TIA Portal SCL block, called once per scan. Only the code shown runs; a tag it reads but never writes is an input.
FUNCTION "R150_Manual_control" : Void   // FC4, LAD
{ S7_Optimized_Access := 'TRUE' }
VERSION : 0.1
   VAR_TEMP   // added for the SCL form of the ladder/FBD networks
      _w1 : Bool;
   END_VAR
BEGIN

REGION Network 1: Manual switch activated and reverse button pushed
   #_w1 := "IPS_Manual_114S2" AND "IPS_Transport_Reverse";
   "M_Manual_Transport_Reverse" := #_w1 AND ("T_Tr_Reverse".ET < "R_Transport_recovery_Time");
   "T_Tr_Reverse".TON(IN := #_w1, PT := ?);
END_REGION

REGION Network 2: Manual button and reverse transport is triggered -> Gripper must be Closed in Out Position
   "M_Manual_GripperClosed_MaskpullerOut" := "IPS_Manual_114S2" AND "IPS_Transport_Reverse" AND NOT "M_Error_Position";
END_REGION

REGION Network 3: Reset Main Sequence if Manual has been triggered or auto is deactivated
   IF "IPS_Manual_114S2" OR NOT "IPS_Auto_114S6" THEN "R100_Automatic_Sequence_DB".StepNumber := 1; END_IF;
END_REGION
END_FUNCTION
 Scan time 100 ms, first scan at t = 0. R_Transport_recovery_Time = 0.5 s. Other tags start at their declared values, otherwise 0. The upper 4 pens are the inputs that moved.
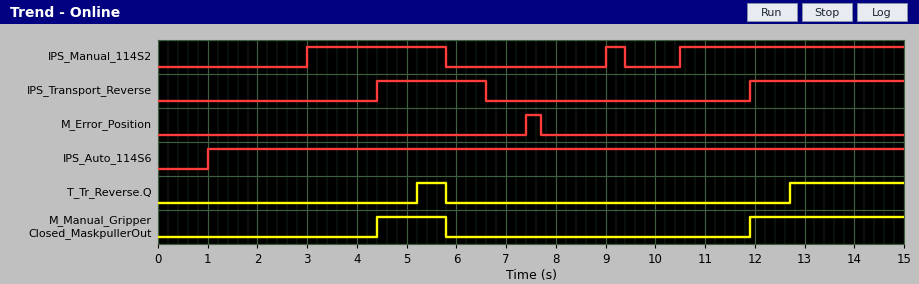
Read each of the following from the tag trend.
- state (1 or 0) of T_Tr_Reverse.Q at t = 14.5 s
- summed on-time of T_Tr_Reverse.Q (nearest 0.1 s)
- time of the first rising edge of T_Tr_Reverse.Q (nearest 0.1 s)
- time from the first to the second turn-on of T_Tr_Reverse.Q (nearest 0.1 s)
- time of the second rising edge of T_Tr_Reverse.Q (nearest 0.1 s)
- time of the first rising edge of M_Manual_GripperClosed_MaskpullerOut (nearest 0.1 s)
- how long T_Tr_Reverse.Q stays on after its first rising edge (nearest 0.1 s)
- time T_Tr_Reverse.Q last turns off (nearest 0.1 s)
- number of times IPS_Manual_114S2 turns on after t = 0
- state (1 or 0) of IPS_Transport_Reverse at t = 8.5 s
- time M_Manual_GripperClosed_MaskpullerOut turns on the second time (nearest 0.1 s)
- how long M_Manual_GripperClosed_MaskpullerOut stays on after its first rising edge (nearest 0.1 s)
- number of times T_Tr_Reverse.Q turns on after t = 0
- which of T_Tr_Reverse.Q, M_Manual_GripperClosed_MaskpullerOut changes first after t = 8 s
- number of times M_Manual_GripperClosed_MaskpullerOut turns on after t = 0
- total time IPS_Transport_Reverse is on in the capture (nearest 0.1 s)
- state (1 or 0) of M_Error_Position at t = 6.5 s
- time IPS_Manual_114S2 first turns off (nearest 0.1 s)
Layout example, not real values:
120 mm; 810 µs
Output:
1; 2.9 s; 5.2 s; 7.5 s; 12.7 s; 4.4 s; 0.6 s; 5.8 s; 3; 0; 11.9 s; 1.4 s; 2; M_Manual_GripperClosed_MaskpullerOut; 2; 5.3 s; 0; 5.8 s
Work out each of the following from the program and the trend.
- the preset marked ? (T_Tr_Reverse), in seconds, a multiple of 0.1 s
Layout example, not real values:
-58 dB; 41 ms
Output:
0.8 s
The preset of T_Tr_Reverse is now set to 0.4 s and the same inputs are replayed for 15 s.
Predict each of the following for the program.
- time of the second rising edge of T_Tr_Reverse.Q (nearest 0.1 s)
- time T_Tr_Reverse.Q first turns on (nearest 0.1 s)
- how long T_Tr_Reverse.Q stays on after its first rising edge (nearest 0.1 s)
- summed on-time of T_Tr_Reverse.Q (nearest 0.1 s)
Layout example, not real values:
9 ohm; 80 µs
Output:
12.3 s; 4.8 s; 1.0 s; 3.7 s
